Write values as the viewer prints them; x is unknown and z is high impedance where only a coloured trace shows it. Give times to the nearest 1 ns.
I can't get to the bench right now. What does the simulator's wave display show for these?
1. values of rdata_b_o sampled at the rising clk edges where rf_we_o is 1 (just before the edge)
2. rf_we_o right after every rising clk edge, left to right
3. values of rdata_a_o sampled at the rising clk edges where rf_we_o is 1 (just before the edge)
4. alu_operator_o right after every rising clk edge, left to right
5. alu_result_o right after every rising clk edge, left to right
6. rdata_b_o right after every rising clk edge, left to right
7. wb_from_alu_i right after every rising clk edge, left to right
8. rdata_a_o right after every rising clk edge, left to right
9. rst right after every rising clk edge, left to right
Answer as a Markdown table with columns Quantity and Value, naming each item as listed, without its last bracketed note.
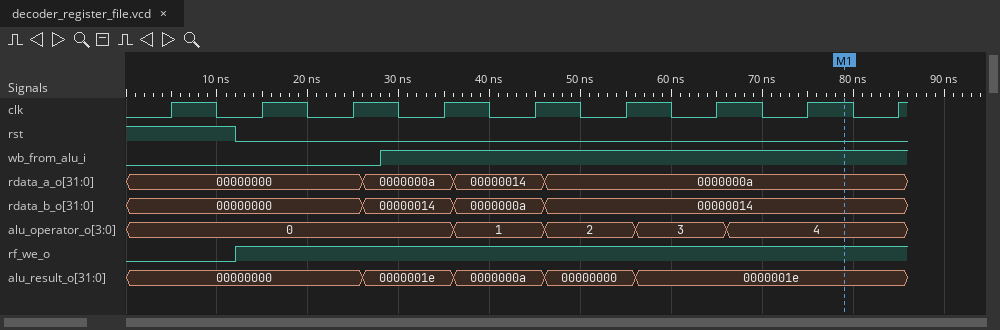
| Quantity | Value |
|---|---|
| values of rdata_b_o sampled at the rising clk edges where rf_we_o is 1 | 00000000, 00000000, 00000014, 0000000a, 00000014, 00000014, 00000014, 00000014 |
| rf_we_o right after every rising clk edge, left to right | 0 1 1 1 1 1 1 1 1 |
| values of rdata_a_o sampled at the rising clk edges where rf_we_o is 1 | 00000000, 00000000, 0000000a, 00000014, 0000000a, 0000000a, 0000000a, 0000000a |
| alu_operator_o right after every rising clk edge, left to right | 0, 0, 0, 0, 1, 2, 3, 4, 4 |
| alu_result_o right after every rising clk edge, left to right | 00000000, 00000000, 00000000, 0000001e, 0000000a, 00000000, 0000001e, 0000001e, 0000001e |
| rdata_b_o right after every rising clk edge, left to right | 00000000, 00000000, 00000000, 00000014, 0000000a, 00000014, 00000014, 00000014, 00000014 |
| wb_from_alu_i right after every rising clk edge, left to right | 0 0 0 1 1 1 1 1 1 |
| rdata_a_o right after every rising clk edge, left to right | 00000000, 00000000, 00000000, 0000000a, 00000014, 0000000a, 0000000a, 0000000a, 0000000a |
| rst right after every rising clk edge, left to right | 1 0 0 0 0 0 0 0 0 |
